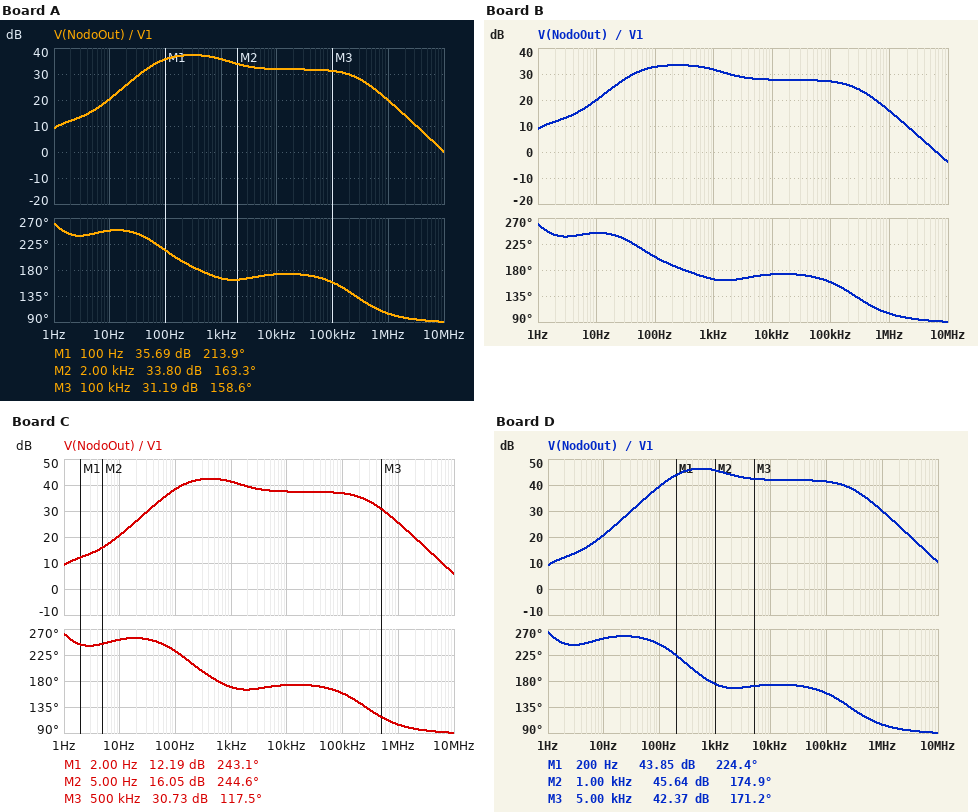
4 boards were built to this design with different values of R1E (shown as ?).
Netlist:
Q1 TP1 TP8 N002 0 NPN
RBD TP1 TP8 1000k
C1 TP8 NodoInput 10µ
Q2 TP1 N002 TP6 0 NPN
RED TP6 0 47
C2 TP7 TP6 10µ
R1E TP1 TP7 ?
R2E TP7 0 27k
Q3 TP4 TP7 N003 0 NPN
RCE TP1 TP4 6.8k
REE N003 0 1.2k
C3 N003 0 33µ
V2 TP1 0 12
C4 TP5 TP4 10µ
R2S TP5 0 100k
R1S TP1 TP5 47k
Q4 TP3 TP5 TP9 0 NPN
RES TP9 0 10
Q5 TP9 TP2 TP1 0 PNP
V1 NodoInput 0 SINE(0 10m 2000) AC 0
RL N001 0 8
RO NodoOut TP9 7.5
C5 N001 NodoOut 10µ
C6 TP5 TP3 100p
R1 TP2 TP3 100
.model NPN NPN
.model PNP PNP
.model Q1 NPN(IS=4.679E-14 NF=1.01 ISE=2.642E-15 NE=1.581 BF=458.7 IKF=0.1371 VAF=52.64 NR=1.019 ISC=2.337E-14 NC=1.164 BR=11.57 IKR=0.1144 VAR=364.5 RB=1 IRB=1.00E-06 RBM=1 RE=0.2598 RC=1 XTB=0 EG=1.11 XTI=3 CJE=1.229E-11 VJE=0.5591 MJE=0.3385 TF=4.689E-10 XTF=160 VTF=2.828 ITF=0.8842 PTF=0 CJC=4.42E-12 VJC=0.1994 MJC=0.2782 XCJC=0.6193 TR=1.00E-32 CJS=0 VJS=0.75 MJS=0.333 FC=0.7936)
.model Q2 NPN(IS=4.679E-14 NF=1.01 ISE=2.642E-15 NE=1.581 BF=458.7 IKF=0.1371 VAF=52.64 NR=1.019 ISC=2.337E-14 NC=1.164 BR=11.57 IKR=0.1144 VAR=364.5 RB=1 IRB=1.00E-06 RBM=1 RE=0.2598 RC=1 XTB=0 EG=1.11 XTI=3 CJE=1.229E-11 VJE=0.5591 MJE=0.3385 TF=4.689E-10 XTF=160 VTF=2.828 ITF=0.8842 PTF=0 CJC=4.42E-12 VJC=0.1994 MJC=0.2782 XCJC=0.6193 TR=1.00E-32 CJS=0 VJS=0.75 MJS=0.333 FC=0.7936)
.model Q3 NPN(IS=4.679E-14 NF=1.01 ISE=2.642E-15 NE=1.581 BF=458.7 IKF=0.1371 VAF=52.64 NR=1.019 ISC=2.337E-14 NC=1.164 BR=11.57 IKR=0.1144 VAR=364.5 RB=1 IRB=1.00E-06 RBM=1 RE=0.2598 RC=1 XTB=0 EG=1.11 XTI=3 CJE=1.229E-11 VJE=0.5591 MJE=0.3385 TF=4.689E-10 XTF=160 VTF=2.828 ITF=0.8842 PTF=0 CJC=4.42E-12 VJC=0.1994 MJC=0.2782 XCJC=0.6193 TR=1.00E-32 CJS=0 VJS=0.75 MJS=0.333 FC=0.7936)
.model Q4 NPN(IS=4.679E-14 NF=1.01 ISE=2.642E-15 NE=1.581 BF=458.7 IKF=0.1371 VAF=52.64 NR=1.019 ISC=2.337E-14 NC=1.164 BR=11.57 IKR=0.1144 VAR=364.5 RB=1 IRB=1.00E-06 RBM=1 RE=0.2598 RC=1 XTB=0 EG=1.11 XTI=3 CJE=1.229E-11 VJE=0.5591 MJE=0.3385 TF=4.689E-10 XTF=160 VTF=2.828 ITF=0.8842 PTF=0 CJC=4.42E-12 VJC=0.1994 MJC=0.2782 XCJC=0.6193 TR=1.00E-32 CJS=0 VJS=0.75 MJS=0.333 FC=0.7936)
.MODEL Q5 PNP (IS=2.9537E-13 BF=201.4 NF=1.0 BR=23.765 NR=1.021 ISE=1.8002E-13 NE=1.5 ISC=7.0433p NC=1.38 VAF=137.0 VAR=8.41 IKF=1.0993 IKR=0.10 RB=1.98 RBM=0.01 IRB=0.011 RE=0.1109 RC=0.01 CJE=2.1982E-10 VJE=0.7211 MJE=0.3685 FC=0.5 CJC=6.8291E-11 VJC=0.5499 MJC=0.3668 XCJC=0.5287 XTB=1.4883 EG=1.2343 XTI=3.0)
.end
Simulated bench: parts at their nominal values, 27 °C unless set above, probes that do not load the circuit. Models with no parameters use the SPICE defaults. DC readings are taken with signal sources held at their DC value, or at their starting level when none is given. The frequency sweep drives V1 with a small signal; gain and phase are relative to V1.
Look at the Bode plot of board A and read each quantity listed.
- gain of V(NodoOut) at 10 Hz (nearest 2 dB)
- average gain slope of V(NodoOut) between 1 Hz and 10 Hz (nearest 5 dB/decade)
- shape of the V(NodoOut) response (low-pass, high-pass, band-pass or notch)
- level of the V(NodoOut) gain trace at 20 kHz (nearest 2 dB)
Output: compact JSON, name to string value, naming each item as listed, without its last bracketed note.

{"gain of V(NodoOut) at 10 Hz": "20 dB", "average gain slope of V(NodoOut) between 1 Hz and 10 Hz": "10 dB/decade", "shape of the V(NodoOut) response": "band-pass", "level of the V(NodoOut) gain trace at 20 kHz": "32 dB"}
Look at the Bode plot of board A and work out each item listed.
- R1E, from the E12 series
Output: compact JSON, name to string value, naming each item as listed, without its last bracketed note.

{"R1E, from the E12 series": "220 kΩ"}
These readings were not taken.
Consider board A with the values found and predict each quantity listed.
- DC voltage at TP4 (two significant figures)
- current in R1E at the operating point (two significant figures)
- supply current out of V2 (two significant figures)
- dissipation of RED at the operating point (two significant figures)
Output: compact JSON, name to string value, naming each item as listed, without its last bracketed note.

{"DC voltage at TP4": "9.4 V", "current in R1E at the operating point": "49 µA", "supply current out of V2": "630 mA", "dissipation of RED at the operating point": "240 mW"}
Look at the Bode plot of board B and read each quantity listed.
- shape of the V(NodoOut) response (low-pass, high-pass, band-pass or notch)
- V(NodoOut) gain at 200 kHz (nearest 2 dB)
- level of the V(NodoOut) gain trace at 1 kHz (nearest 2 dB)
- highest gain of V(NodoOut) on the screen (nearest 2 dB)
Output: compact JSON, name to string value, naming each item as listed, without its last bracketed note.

{"shape of the V(NodoOut) response": "band-pass", "V(NodoOut) gain at 200 kHz": "26 dB", "level of the V(NodoOut) gain trace at 1 kHz": "32 dB", "highest gain of V(NodoOut) on the screen": "34 dB"}
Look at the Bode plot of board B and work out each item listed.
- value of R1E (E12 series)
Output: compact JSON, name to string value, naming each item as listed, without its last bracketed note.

{"value of R1E": "270 kΩ"}
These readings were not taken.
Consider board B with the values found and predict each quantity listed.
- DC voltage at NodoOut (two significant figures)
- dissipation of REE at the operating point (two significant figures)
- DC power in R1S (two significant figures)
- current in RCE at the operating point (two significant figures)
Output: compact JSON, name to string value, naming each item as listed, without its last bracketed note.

{"DC voltage at NodoOut": "5.6 V", "dissipation of REE at the operating point": "72 µW", "DC power in R1S": "670 µW", "current in RCE at the operating point": "240 µA"}
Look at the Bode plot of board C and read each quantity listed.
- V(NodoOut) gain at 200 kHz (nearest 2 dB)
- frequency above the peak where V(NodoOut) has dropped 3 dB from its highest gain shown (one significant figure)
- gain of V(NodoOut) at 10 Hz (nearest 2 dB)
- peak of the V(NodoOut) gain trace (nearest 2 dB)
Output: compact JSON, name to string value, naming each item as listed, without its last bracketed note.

{"V(NodoOut) gain at 200 kHz": "36 dB", "frequency above the peak where V(NodoOut) has dropped 3 dB from its highest gain shown": "2 kHz", "gain of V(NodoOut) at 10 Hz": "20 dB", "peak of the V(NodoOut) gain trace": "42 dB"}
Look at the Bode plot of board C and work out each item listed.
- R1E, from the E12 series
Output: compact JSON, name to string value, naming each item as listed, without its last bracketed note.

{"R1E, from the E12 series": "150 kΩ"}
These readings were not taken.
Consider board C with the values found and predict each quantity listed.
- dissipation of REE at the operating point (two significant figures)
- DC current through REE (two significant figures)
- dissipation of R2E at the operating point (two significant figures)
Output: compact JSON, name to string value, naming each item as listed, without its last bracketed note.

{"dissipation of REE at the operating point": "670 µW", "DC current through REE": "750 µA", "dissipation of R2E at the operating point": "100 µW"}
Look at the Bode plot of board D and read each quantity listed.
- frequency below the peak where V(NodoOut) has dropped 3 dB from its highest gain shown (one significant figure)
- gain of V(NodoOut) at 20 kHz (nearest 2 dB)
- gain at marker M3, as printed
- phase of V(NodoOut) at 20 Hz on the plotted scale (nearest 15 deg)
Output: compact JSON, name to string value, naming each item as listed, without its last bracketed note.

{"frequency below the peak where V(NodoOut) has dropped 3 dB from its highest gain shown": "200 Hz", "gain of V(NodoOut) at 20 kHz": "42 dB", "gain at marker M3, as printed": "42.37 dB", "phase of V(NodoOut) at 20 Hz on the plotted scale": "255 deg"}
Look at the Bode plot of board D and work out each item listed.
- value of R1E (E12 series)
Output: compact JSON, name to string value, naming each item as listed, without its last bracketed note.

{"value of R1E": "100 kΩ"}
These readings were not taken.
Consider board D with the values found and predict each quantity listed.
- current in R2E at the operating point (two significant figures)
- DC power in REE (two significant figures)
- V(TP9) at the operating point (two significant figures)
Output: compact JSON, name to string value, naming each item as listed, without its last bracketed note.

{"current in R2E at the operating point": "85 µA", "DC power in REE": "1.9 mW", "V(TP9) at the operating point": "5.6 V"}
